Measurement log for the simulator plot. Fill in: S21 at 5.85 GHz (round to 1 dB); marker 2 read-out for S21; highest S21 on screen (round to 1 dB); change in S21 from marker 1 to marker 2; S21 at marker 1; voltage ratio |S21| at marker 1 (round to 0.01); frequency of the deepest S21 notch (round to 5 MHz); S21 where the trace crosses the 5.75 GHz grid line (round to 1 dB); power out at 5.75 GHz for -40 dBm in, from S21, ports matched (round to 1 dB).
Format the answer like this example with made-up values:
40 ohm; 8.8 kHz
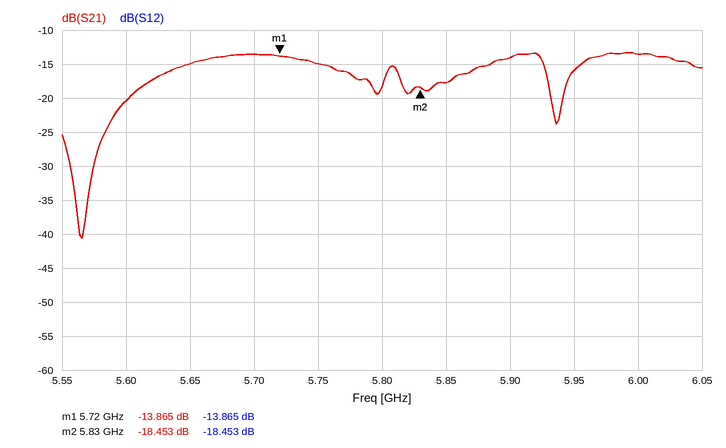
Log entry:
-18 dB; -18.453 dB; -13 dB; -4.588 dB; -13.865 dB; 0.20; 5.565 GHz; -15 dB; -55 dBm
